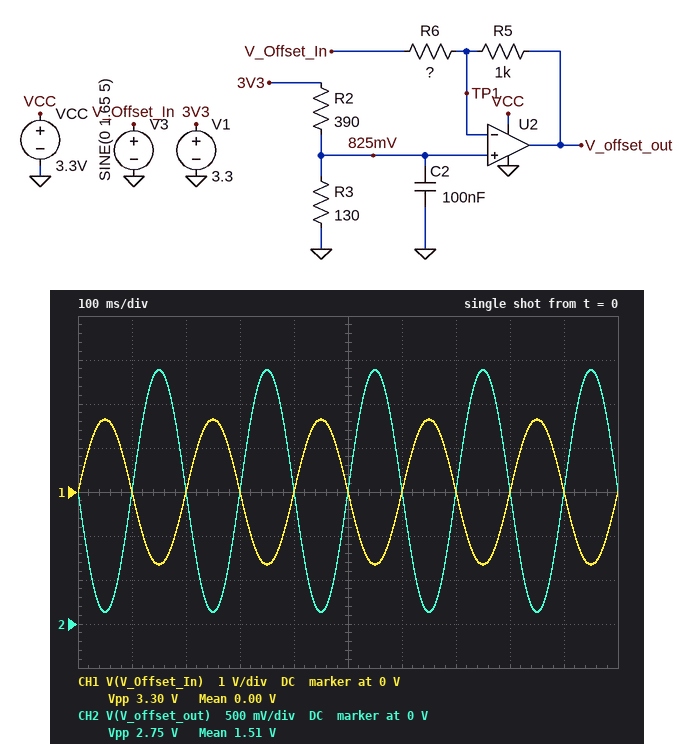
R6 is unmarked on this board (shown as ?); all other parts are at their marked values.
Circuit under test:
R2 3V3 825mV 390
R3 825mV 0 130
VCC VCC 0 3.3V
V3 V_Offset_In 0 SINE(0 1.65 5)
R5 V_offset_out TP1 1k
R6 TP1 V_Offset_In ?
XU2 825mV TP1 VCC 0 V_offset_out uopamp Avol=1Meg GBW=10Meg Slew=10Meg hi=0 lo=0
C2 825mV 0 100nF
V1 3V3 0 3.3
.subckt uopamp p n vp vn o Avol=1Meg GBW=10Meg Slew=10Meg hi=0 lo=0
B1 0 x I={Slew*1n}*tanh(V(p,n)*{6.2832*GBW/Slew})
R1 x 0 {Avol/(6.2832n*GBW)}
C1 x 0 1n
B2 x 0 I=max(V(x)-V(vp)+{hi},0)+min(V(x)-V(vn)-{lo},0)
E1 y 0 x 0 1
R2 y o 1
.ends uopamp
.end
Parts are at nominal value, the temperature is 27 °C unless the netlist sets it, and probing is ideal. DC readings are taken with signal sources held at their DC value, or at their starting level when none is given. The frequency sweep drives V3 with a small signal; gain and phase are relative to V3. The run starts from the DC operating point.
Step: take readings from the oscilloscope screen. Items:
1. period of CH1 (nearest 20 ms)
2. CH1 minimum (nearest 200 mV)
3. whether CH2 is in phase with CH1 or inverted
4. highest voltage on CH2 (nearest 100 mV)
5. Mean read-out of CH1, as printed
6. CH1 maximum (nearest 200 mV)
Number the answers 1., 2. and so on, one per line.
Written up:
1. 200 ms
2. -1.6 V
3. inverted
4. 2.9 V
5. 0.00 V
6. 1.6 V
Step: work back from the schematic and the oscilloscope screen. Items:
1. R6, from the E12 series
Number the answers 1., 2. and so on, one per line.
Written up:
1. 1.2 kΩ
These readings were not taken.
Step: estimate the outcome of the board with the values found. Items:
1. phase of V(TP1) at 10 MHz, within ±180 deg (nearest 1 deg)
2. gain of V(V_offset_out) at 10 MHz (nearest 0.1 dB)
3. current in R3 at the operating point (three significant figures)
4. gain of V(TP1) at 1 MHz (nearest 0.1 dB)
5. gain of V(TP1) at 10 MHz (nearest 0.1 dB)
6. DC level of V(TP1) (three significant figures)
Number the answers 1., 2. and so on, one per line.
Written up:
1. 29 deg
2. -8.0 dB
3. 6.35 mA
4. -21.7 dB
5. -8.0 dB
6. 825 mV
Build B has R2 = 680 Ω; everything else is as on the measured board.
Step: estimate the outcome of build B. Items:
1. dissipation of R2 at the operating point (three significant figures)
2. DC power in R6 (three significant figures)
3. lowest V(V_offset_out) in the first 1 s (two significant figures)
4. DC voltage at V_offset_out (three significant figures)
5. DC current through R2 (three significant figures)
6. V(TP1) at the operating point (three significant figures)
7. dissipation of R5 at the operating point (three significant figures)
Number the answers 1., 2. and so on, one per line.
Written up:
1. 11.3 mW
2. 234 µW
3. -8.0 mV
4. 971 mV
5. 4.07 mA
6. 530 mV
7. 195 µW
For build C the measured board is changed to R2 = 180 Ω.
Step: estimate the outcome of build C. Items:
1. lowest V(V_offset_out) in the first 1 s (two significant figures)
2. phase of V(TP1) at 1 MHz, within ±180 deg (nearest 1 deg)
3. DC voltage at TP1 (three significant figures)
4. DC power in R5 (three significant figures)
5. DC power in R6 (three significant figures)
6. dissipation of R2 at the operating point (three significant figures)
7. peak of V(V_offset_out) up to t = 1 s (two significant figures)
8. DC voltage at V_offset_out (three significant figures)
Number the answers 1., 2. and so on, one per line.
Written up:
1. 1.2 V
2. 80 deg
3. 1.38 V
4. 1.33 mW
5. 1.60 mW
6. 20.4 mW
7. 3.3 V
8. 2.54 V
